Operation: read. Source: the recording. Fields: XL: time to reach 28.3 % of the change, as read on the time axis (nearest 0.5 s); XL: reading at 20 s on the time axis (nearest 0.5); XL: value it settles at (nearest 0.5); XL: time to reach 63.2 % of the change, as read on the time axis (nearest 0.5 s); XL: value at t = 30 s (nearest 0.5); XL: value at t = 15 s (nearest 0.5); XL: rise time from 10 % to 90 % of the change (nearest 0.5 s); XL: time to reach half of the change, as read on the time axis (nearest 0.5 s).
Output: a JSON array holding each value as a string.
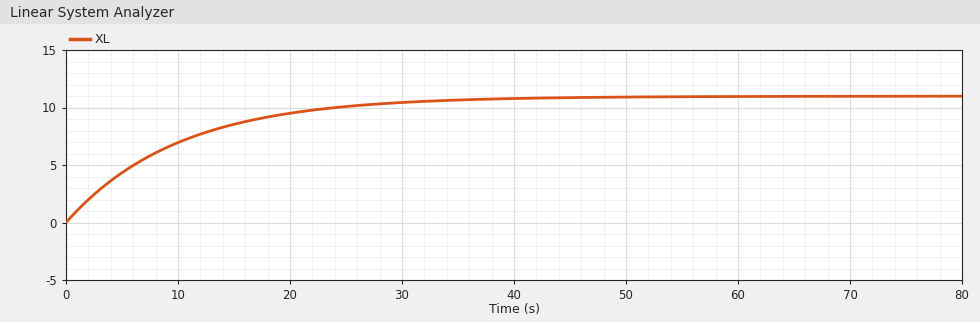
["3.5 s", "9.5", "11.0", "10.0 s", "10.5", "8.5", "22.0 s", "7.0 s"]
